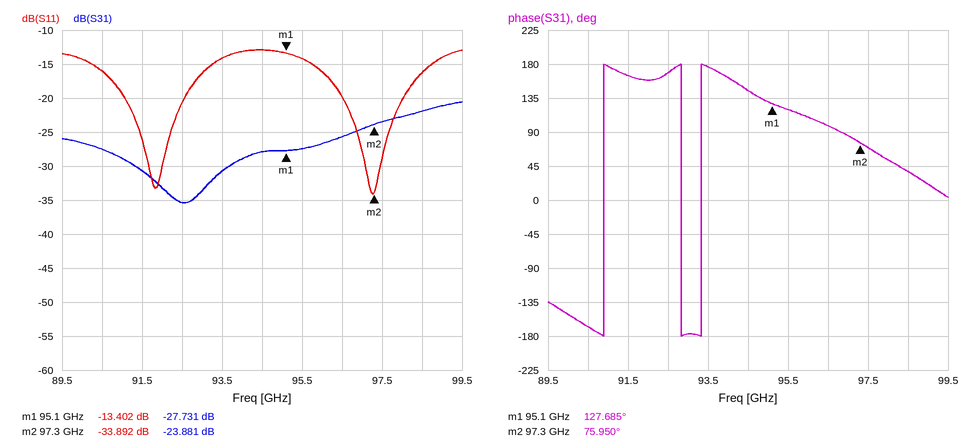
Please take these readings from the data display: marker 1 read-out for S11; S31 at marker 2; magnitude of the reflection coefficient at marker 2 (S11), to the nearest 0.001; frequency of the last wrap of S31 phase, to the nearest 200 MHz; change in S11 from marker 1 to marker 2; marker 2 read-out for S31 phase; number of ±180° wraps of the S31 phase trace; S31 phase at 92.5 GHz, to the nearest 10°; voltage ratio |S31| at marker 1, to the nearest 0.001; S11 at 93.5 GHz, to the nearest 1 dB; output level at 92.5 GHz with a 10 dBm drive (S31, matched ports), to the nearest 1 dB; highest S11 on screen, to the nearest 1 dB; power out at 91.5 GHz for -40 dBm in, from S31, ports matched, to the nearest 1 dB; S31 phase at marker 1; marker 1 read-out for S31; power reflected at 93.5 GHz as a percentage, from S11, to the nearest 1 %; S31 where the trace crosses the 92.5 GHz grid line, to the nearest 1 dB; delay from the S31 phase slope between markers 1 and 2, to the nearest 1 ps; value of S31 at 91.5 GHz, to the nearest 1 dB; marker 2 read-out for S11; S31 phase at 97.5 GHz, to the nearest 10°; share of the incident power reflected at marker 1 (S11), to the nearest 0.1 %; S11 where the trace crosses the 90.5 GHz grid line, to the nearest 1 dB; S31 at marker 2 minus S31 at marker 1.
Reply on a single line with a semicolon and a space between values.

-13.402 dB; -23.881 dB; 0.020; 93.4 GHz; -20.490 dB; 75.950°; 3; 170°; 0.041; -14 dB; -25 dBm; -13 dB; -71 dBm; 127.685°; -27.731 dB; 4 %; -35 dB; 65 ps; -31 dB; -33.892 dB; 70°; 4.6 %; -16 dB; 3.850 dB
